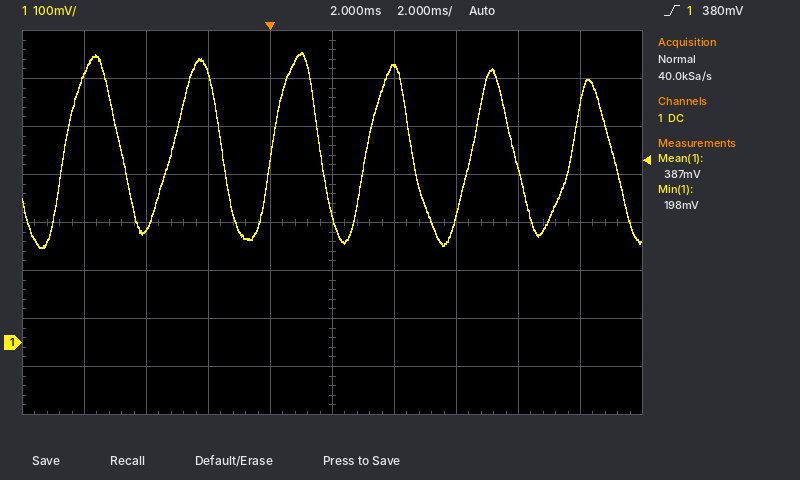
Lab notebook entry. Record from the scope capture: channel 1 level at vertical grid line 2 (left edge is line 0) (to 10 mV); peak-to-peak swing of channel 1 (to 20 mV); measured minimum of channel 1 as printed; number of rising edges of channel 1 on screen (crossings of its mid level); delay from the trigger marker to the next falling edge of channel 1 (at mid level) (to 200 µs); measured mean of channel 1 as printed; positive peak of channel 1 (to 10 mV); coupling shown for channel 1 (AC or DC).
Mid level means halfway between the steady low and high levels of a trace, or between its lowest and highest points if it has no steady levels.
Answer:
240 mV
400 mV
198 mV
6
1.6 ms
387 mV
600 mV
DC
